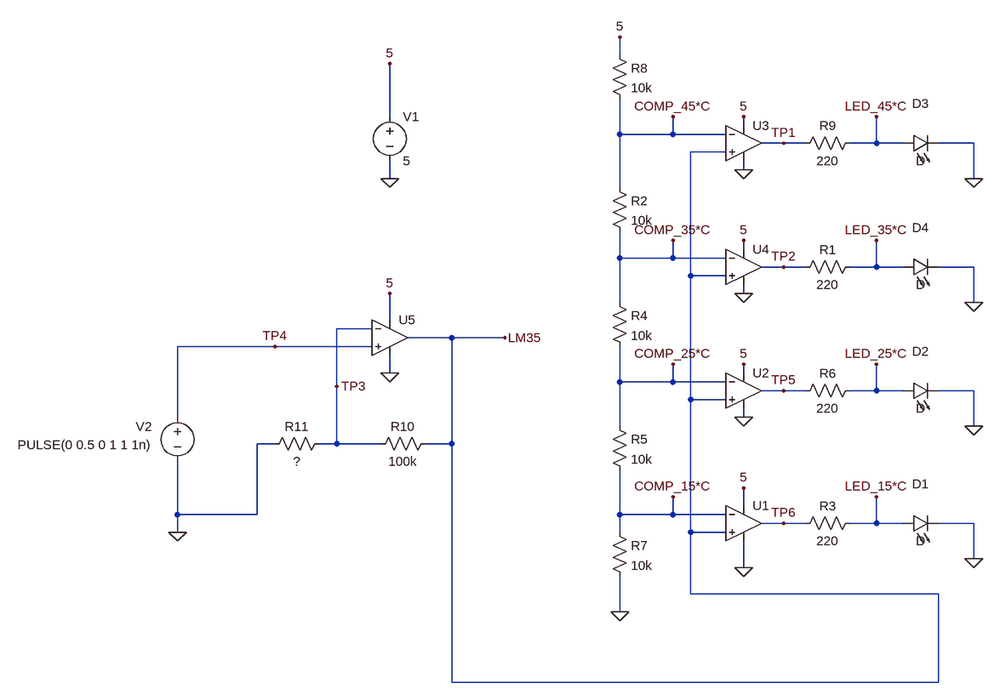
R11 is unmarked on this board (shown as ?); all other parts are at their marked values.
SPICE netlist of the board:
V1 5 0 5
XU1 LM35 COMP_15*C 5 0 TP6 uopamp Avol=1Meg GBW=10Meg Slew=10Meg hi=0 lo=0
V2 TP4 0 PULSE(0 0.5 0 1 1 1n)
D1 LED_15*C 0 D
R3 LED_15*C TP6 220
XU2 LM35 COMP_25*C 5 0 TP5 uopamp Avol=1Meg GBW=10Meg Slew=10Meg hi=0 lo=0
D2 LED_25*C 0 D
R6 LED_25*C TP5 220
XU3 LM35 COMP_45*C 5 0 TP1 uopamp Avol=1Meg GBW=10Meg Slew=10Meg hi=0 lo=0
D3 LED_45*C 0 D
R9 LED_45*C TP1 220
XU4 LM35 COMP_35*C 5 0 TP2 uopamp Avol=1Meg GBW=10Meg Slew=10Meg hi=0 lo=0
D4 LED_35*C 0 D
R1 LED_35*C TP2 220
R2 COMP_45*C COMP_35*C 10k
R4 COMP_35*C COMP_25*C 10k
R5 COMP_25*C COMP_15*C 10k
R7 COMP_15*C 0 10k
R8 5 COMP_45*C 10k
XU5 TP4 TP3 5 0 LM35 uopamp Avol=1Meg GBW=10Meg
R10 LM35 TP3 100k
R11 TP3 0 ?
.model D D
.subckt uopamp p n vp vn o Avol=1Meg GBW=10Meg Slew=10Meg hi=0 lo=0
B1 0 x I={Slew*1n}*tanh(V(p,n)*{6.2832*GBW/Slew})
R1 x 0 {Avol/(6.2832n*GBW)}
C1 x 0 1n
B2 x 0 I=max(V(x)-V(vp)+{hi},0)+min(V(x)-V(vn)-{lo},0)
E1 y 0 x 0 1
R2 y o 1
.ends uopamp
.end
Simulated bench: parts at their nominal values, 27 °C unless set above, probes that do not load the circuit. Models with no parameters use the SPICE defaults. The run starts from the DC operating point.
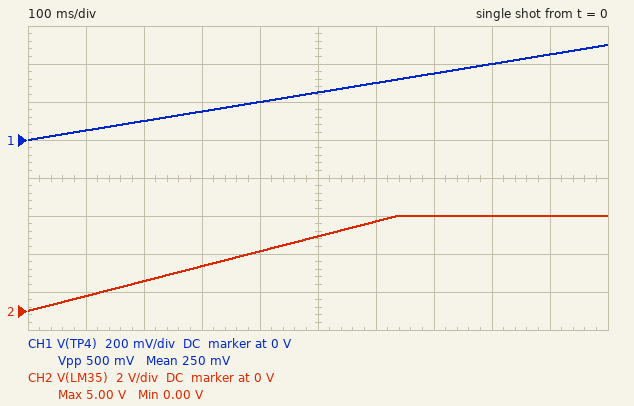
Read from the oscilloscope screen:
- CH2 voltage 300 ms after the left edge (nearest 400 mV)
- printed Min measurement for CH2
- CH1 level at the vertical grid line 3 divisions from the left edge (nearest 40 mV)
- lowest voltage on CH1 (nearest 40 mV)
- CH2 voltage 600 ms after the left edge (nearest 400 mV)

2.4 V
0.00 V
160 mV
0 V
4.8 V
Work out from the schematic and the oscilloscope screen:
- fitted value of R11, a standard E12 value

6.8 kΩ
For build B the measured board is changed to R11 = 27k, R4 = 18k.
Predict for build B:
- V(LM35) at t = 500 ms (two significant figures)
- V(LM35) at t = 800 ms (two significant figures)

1.2 V
1.9 V
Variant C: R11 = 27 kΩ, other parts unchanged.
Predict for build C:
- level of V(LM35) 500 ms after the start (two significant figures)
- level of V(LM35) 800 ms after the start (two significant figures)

1.2 V
1.9 V
